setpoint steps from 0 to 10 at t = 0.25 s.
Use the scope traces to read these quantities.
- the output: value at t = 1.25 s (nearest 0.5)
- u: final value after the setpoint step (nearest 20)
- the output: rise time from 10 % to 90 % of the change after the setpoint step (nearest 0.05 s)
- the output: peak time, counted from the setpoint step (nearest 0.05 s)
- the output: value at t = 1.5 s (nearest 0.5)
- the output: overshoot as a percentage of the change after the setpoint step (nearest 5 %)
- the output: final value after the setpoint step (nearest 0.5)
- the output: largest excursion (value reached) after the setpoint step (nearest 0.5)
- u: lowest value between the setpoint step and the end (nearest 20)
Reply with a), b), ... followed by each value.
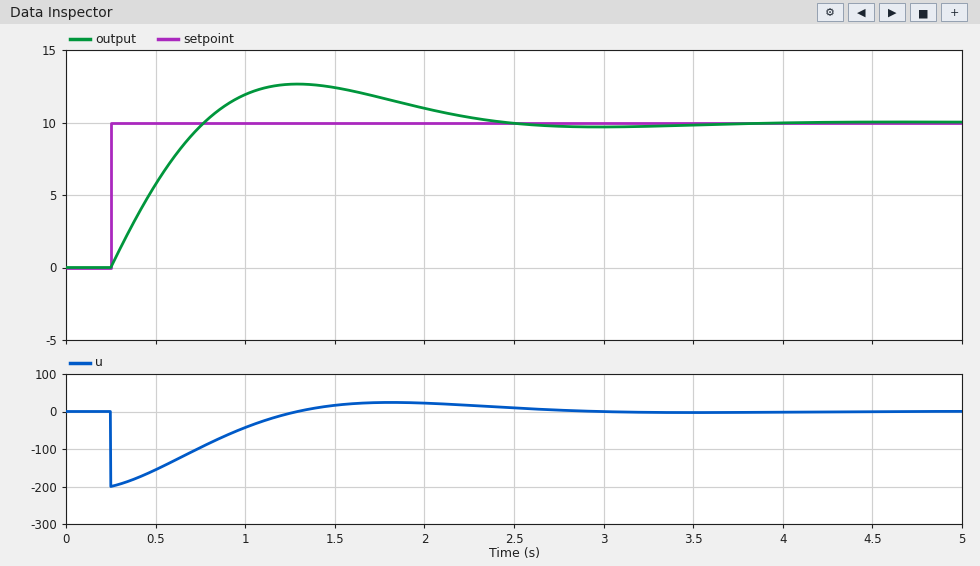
a) 12.5
b) 0
c) 0.40 s
d) 1.05 s
e) 12.5
f) 25 %
g) 10.0
h) 12.5
i) -200
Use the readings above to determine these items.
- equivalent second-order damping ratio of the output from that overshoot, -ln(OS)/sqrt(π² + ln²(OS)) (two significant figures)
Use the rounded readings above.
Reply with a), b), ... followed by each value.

a) 0.40
